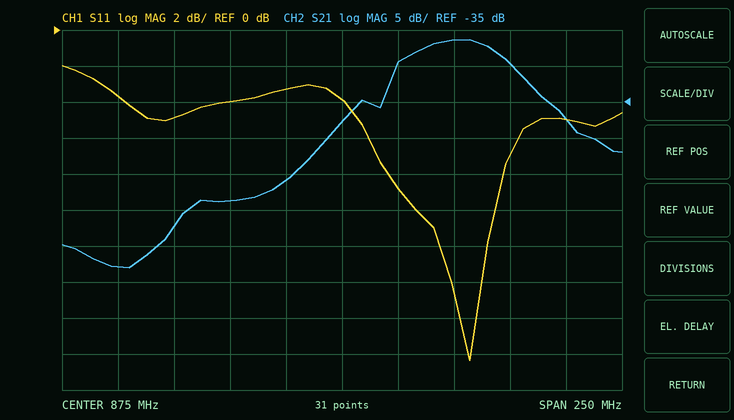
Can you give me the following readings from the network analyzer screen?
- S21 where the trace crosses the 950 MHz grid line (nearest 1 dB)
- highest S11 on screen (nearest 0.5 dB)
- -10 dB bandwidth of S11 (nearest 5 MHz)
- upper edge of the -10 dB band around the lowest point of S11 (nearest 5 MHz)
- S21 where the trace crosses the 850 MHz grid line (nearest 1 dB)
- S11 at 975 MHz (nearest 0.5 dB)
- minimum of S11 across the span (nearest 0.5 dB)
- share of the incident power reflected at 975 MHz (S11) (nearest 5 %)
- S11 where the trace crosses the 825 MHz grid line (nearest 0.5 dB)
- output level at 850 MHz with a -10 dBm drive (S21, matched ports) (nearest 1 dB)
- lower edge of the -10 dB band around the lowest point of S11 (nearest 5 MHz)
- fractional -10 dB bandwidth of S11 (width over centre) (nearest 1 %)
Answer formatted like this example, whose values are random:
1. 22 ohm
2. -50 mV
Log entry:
1. -30 dB
2. -2.0 dB
3. 35 MHz
4. 945 MHz
5. -46 dB
6. -5.0 dB
7. -18.5 dB
8. 30 %
9. -4.0 dB
10. -56 dBm
11. 910 MHz
12. 4 %
